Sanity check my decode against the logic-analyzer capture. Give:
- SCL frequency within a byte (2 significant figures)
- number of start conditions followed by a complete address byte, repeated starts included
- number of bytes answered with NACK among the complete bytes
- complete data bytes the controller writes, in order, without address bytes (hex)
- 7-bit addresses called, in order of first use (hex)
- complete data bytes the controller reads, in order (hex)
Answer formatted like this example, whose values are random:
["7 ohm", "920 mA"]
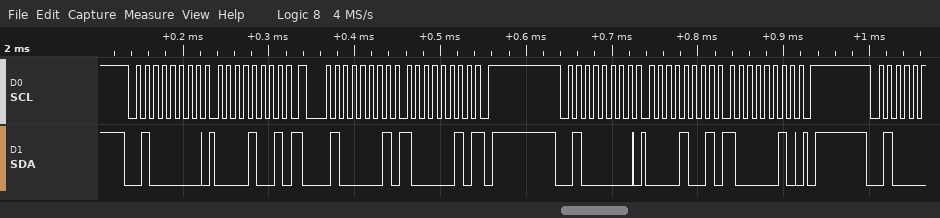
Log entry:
["100 kHz", "3", "1", "09 09 82", "0x20", "82"]
